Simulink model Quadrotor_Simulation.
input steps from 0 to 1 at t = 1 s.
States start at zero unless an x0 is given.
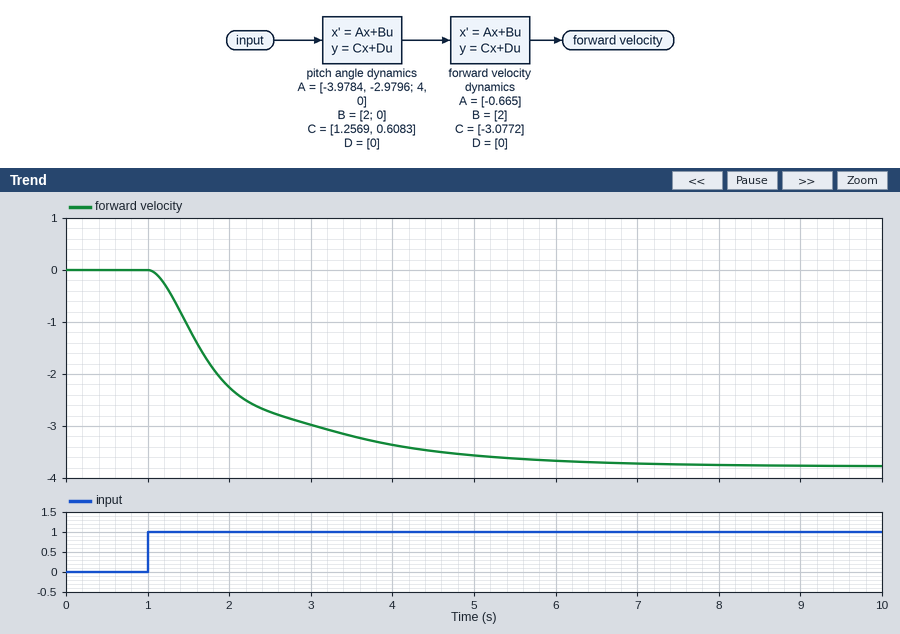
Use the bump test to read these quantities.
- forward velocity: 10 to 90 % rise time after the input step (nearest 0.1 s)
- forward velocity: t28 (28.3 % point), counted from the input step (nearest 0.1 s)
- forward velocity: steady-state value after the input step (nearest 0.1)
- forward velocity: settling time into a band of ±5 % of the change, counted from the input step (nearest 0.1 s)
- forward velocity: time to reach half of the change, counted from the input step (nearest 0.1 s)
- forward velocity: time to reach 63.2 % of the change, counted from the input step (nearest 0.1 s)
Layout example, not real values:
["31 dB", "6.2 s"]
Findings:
["2.9 s", "0.5 s", "-3.8", "4.2 s", "0.8 s", "1.1 s"]
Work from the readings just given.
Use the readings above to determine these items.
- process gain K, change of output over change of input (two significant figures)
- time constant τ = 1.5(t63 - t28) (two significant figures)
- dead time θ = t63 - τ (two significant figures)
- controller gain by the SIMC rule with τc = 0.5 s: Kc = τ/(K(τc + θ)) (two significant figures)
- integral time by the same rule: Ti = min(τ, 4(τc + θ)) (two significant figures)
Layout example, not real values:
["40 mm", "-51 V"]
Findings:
["-3.8", "0.90 s", "0.20 s", "-0.34", "0.90 s"]
